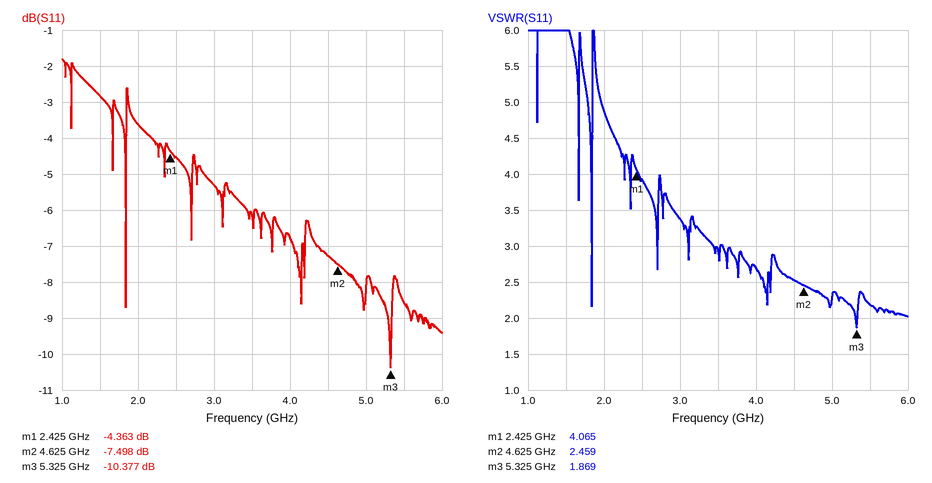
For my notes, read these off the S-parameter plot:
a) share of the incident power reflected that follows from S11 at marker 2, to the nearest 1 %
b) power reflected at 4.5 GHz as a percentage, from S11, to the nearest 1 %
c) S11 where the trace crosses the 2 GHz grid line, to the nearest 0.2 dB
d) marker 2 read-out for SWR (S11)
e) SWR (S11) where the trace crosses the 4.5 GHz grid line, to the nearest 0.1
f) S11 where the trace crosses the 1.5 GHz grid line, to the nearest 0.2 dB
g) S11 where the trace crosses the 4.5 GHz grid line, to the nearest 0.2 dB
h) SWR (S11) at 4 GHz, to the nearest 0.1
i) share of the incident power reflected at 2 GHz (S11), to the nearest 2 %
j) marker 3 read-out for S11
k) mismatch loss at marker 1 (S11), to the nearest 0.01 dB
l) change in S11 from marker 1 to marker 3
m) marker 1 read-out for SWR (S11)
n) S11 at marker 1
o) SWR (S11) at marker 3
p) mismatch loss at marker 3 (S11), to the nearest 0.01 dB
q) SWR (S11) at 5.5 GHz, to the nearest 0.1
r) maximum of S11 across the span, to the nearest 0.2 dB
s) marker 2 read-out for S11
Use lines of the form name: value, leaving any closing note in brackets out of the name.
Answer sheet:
share of the incident power reflected that follows from S11 at marker 2, to the nearest 1 %: 18 %
power reflected at 4.5 GHz as a percentage, from S11, to the nearest 1 %: 19 %
S11 where the trace crosses the 2 GHz grid line, to the nearest 0.2 dB: -3.6 dB
marker 2 read-out for SWR: 2.459
SWR (S11) where the trace crosses the 4.5 GHz grid line, to the nearest 0.1: 2.5
S11 where the trace crosses the 1.5 GHz grid line, to the nearest 0.2 dB: -2.8 dB
S11 where the trace crosses the 4.5 GHz grid line, to the nearest 0.2 dB: -7.2 dB
SWR (S11) at 4 GHz, to the nearest 0.1: 2.7
share of the incident power reflected at 2 GHz (S11), to the nearest 2 %: 44 %
marker 3 read-out for S11: -10.377 dB
mismatch loss at marker 1 (S11), to the nearest 0.01 dB: 1.98 dB
change in S11 from marker 1 to marker 3: -6.014 dB
marker 1 read-out for SWR: 4.065
S11 at marker 1: -4.363 dB
SWR (S11) at marker 3: 1.869
mismatch loss at marker 3 (S11), to the nearest 0.01 dB: 0.42 dB
SWR (S11) at 5.5 GHz, to the nearest 0.1: 2.2
maximum of S11 across the span, to the nearest 0.2 dB: -1.8 dB
marker 2 read-out for S11: -7.498 dB
